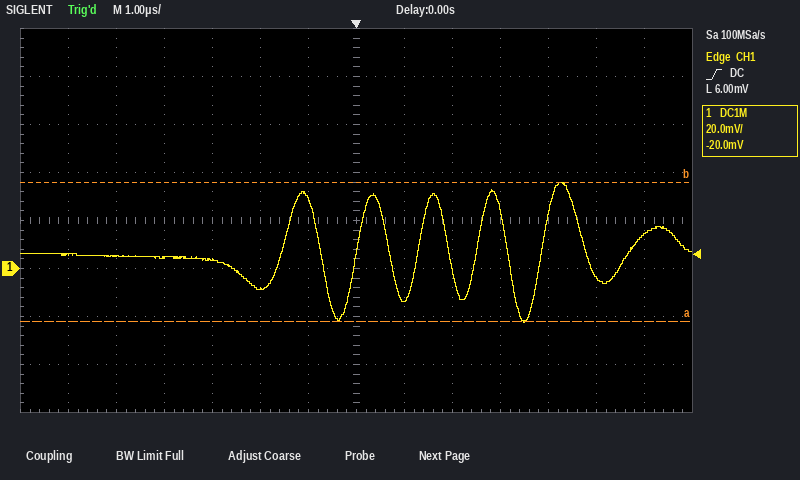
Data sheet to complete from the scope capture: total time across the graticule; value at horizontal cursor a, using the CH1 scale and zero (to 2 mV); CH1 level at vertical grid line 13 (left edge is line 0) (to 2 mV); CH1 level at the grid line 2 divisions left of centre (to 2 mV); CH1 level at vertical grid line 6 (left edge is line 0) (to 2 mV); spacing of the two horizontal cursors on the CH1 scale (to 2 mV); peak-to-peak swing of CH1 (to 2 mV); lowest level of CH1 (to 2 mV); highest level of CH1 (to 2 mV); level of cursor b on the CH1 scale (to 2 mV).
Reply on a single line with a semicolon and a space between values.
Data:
14 µs; -22 mV; 14 mV; -8 mV; 28 mV; 58 mV; 58 mV; -22 mV; 36 mV; 36 mV
